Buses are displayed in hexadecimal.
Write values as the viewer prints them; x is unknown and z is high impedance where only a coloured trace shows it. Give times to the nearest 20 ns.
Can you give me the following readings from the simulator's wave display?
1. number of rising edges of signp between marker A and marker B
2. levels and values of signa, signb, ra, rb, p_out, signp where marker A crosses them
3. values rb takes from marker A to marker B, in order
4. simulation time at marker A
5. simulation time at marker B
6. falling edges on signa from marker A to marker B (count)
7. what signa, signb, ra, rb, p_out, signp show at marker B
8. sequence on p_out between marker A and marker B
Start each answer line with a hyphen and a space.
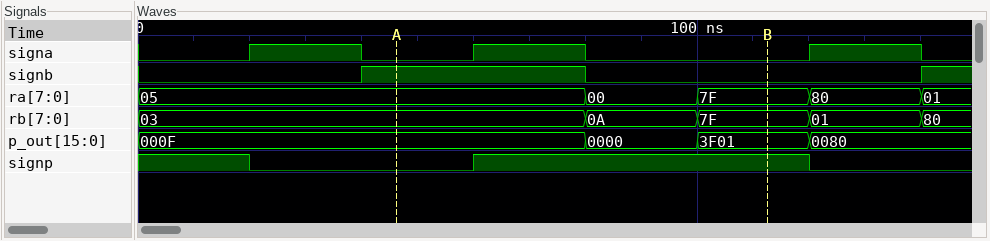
- 1
- signa=0, signb=1, ra=05, rb=03, p_out=000F, signp=0
- 03, 0A, 7F
- 40 ns
- 120 ns
- 1
- signa=0, signb=0, ra=7F, rb=7F, p_out=3F01, signp=1
- 000F, 0000, 3F01
